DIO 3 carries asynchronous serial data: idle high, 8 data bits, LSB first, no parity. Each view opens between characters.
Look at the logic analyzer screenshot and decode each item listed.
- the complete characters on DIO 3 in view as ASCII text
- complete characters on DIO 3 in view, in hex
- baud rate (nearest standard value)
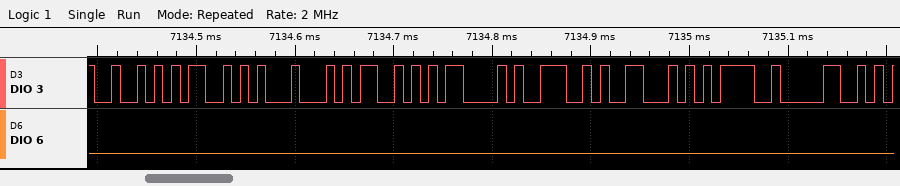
"RSDSCNF=0"
52, 53, 44, 53, 43, 4E, 46, 3D, 30
115200 baud
